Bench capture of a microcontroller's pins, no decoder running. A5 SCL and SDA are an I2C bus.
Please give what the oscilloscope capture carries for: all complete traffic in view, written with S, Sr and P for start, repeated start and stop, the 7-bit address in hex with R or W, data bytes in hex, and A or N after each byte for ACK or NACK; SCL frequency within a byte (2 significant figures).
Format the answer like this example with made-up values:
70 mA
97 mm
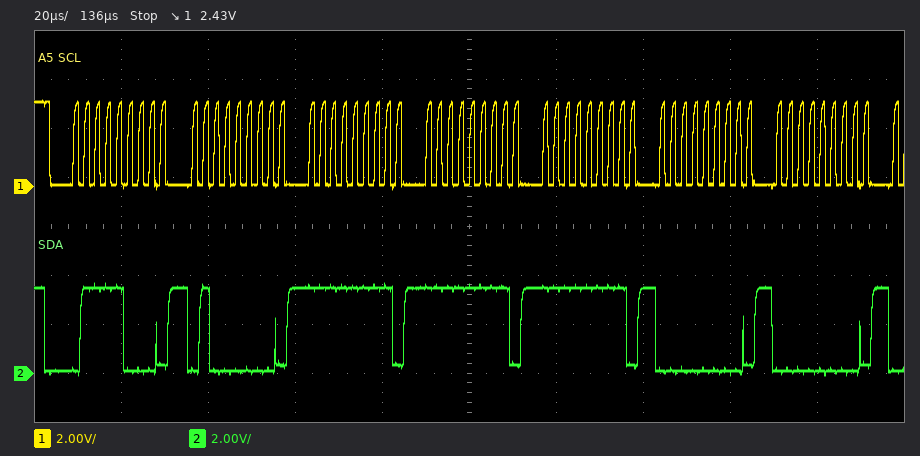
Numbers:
S 3CW A 40 A FF A FF A FF A 00 A 00 A
400 kHz
